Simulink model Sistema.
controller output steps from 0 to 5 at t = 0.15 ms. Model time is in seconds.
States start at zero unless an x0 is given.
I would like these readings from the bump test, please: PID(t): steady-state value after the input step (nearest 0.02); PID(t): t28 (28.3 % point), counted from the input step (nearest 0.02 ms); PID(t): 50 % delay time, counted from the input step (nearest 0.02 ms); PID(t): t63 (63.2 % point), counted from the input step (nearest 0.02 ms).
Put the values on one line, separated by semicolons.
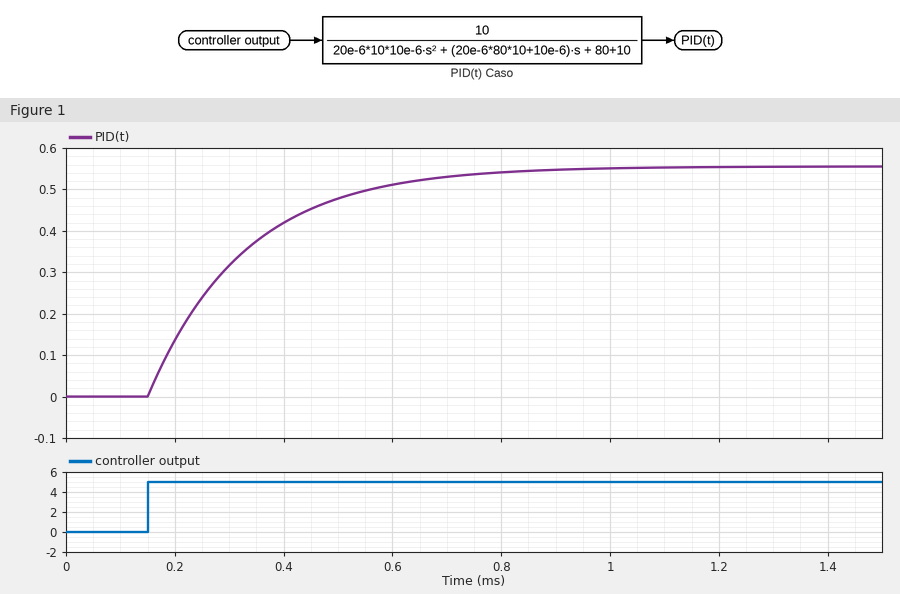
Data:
0.56; 0.06 ms; 0.12 ms; 0.18 ms
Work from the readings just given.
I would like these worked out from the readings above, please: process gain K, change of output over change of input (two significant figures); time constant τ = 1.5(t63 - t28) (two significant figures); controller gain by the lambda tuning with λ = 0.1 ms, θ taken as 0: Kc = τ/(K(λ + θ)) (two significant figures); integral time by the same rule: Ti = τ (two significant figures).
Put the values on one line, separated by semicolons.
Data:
0.11; 0.18 ms; 16; 0.18 ms
